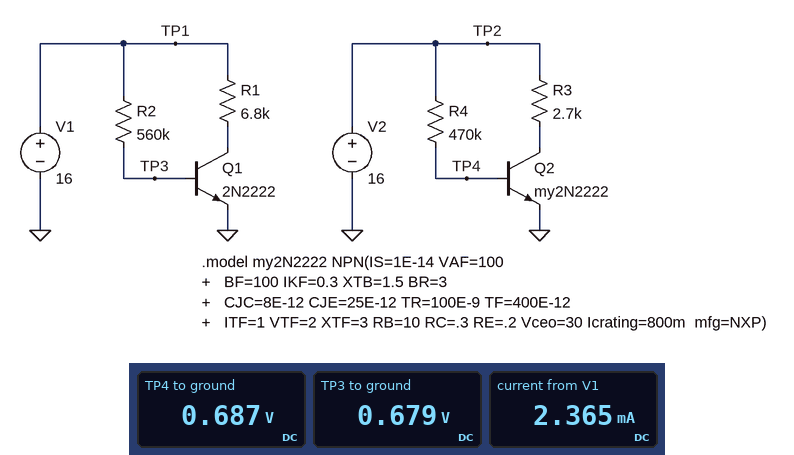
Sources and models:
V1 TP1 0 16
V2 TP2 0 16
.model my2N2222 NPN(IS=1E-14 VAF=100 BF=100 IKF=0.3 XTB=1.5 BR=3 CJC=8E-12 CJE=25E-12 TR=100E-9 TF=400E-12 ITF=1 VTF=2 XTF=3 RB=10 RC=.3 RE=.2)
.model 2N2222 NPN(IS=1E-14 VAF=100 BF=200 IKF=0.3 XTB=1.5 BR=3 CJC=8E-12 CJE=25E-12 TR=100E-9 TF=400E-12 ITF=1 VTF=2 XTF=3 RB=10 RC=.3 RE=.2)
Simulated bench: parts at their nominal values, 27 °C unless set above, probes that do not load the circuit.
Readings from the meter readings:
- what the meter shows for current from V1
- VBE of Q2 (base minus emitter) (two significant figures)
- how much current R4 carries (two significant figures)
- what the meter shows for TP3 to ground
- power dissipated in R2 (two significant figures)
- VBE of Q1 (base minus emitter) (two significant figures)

2.365 mA
690 mV
33 µA
0.679 V
420 µW
680 mV
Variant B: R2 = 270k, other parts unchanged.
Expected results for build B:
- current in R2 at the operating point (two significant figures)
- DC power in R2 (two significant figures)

57 µA
870 µW
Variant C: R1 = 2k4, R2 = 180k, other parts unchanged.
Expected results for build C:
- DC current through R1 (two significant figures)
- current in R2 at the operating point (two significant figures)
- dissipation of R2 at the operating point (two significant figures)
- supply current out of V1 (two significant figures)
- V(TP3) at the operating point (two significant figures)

6.6 mA
85 µA
1.3 mW
6.7 mA
710 mV
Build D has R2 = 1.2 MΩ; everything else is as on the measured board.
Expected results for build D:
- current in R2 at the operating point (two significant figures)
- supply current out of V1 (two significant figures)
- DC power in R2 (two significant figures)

13 µA
2.3 mA
200 µW
